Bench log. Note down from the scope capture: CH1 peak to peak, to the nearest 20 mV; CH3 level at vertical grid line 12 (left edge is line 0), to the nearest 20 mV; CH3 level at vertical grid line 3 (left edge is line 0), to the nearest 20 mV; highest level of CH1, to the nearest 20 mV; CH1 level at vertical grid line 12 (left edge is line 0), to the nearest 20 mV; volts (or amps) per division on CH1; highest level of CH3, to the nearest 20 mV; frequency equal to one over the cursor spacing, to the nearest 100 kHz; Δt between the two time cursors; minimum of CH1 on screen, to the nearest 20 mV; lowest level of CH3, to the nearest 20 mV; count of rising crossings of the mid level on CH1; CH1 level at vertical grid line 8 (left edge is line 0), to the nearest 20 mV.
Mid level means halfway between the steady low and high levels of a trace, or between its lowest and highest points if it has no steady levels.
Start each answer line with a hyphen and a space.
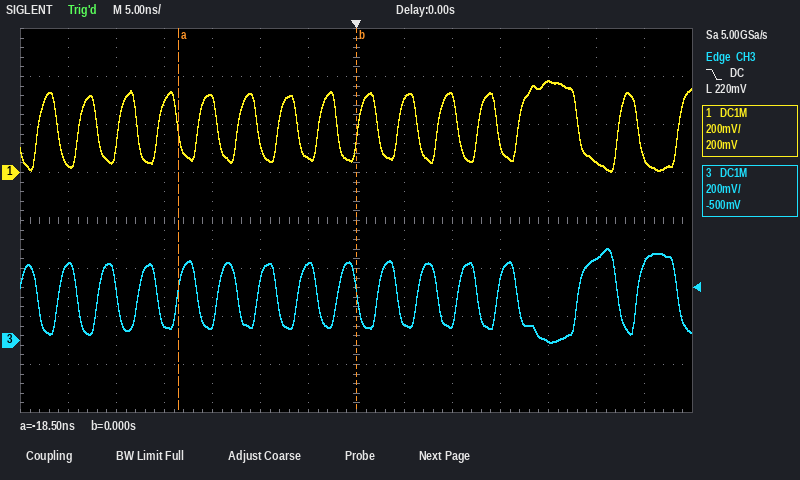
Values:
- 380 mV
- 340 mV
- 60 mV
- 380 mV
- 40 mV
- 200 mV
- 380 mV
- 54.1 MHz
- 18.5 ns
- 0 mV
- 0 mV
- 15
- 300 mV
